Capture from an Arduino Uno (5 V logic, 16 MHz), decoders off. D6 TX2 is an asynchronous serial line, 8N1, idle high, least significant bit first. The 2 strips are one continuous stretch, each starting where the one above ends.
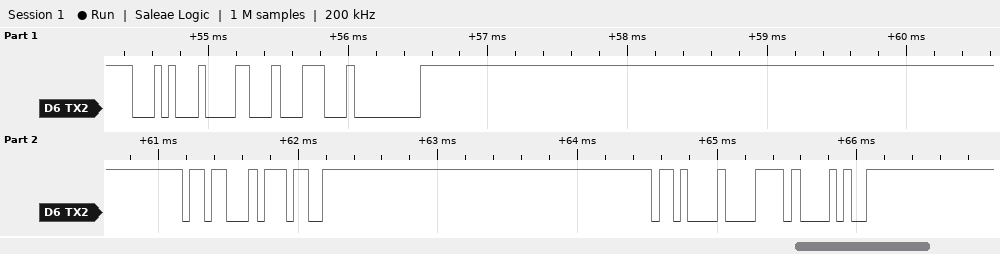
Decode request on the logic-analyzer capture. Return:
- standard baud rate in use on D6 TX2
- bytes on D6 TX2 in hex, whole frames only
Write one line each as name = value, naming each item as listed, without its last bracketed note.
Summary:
standard baud rate in use on D6 TX2 = 19200 baud
bytes on D6 TX2 in hex, whole frames only = 0x14 0x18 0x1C 0x00 0x1B 0x37 0x0B 0x78 0x28
